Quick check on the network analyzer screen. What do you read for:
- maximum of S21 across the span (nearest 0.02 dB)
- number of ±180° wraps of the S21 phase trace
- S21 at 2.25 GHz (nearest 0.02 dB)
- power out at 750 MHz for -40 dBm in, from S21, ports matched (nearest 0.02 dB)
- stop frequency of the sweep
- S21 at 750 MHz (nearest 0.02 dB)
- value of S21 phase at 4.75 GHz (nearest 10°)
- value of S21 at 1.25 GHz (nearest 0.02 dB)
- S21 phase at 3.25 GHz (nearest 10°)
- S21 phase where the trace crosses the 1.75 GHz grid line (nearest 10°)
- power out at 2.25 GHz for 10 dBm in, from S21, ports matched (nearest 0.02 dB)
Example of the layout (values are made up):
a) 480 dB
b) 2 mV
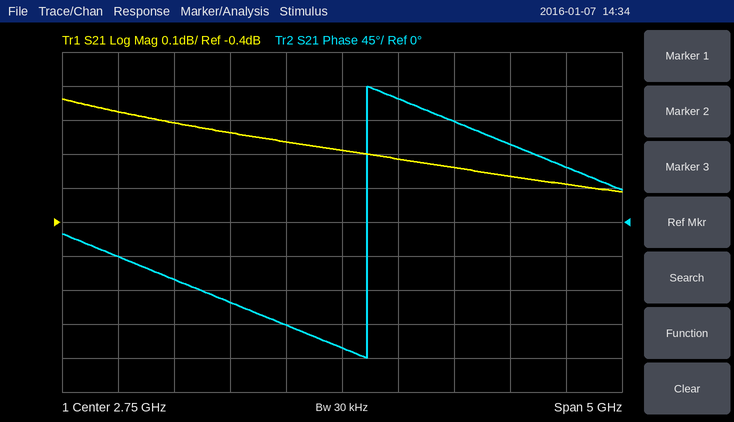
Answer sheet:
a) -0.04 dB
b) 1
c) -0.16 dB
d) -40.08 dBm
e) 5.25 GHz
f) -0.08 dB
g) 70°
h) -0.10 dB
i) 160°
j) -110°
k) 9.84 dBm
